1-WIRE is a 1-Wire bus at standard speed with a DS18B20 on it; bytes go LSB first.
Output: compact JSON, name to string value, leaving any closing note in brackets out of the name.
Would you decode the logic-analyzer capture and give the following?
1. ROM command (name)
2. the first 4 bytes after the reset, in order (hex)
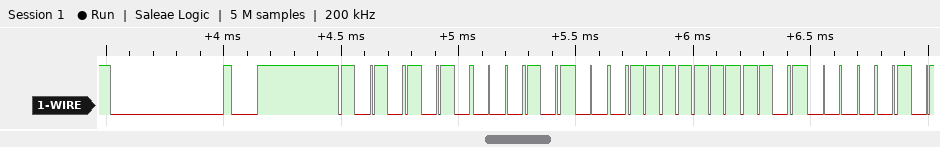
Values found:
{"ROM command": "Match ROM", "the first 4 bytes after the reset, in order": "55 28 FE 0B"}
